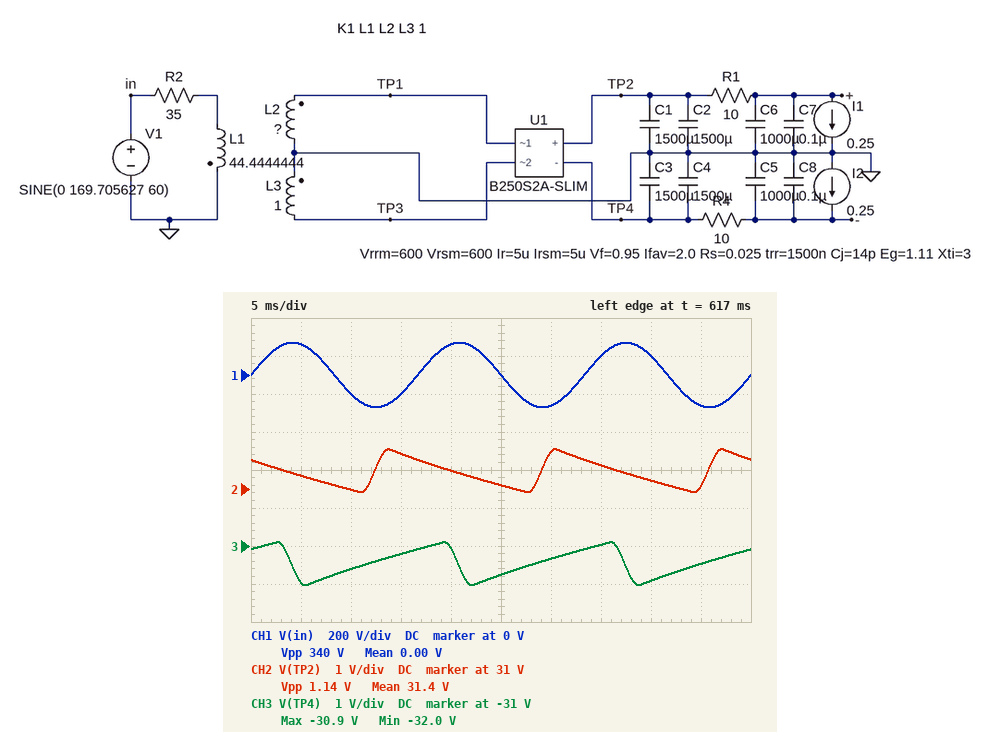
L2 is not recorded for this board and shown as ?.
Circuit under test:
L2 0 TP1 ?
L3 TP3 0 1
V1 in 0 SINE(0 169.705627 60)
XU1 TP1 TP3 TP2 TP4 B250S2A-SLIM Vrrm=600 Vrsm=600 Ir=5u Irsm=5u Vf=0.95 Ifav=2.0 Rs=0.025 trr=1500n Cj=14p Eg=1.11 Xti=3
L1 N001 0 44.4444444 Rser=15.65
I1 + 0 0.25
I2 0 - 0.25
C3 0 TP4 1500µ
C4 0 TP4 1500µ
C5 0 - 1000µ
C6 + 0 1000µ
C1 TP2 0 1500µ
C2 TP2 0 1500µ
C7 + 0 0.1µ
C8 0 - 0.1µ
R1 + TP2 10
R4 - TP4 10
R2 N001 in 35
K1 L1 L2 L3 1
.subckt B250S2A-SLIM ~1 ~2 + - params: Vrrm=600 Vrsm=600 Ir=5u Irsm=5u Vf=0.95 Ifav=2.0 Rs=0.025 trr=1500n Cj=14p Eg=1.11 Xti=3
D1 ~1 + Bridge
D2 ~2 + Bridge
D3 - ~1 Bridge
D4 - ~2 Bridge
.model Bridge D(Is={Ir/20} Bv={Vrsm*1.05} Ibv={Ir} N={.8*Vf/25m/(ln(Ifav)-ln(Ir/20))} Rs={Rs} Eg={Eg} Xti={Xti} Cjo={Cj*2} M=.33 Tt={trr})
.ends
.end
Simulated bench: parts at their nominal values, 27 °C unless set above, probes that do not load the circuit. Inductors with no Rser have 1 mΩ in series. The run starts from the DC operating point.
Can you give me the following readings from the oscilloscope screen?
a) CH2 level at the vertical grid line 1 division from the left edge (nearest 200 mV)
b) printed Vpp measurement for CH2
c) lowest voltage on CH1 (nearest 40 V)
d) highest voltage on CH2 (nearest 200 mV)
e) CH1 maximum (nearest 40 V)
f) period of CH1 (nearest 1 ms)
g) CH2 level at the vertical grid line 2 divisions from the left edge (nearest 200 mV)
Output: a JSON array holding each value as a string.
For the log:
["31.4 V", "1.14 V", "-160 V", "32.0 V", "160 V", "17 ms", "31.0 V"]
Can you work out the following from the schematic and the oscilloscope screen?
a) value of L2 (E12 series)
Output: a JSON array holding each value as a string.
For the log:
["2.2 H"]
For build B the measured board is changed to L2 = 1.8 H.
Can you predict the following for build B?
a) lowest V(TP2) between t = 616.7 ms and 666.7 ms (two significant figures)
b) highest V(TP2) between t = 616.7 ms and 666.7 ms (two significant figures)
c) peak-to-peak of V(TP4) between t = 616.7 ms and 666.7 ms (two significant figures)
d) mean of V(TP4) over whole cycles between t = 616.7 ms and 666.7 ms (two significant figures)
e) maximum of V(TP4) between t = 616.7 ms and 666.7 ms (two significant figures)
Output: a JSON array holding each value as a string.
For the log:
["28 V", "29 V", "1.1 V", "-29 V", "-28 V"]
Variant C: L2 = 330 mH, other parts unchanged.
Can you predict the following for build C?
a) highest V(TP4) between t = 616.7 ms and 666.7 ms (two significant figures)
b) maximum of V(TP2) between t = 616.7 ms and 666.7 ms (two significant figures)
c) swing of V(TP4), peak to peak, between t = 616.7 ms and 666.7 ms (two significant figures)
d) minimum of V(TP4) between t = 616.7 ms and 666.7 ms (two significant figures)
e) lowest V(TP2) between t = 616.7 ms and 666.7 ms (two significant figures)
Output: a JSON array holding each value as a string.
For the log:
["-21 V", "22 V", "1.2 V", "-22 V", "21 V"]
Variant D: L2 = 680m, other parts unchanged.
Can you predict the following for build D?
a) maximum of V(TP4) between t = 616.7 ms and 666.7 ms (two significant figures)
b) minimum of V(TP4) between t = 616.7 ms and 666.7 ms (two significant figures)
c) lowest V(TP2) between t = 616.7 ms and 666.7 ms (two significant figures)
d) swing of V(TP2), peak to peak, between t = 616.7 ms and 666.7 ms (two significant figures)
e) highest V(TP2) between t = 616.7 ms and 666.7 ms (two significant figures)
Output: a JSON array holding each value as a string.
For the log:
["-21 V", "-22 V", "21 V", "1.2 V", "22 V"]
